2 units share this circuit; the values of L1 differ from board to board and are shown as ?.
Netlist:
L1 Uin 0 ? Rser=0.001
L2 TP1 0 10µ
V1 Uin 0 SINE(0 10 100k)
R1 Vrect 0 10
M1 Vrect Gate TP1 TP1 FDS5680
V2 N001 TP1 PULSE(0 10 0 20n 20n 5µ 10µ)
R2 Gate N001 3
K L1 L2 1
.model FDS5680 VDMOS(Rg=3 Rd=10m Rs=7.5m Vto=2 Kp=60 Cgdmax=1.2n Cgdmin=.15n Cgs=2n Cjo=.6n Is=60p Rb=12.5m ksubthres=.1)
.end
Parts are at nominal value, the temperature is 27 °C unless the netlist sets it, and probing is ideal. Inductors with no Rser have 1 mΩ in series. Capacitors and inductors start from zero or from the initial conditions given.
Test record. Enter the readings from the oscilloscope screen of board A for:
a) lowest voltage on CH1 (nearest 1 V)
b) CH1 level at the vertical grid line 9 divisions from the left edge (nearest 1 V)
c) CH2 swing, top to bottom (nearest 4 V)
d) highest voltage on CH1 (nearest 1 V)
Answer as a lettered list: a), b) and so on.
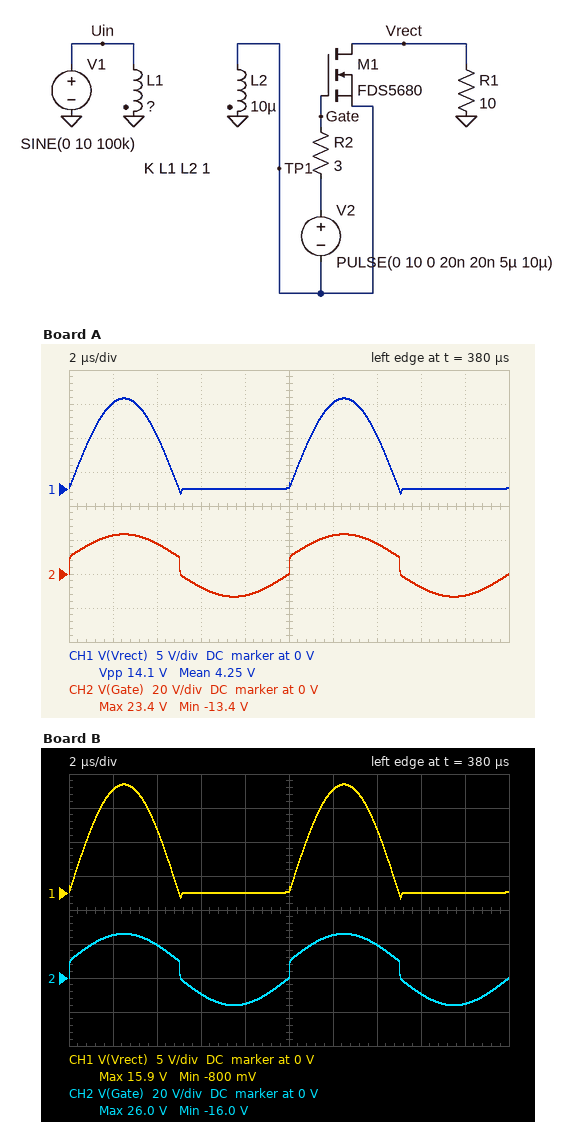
a) -1 V
b) 0 V
c) 36 V
d) 13 V
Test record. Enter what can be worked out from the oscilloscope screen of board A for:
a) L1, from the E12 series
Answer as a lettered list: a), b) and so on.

a) 5.6 µH
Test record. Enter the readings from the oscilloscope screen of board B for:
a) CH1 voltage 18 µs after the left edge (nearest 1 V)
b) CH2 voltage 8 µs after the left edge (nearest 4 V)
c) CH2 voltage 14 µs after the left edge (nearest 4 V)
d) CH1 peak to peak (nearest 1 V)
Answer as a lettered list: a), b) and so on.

a) 0 V
b) -16 V
c) 20 V
d) 17 V
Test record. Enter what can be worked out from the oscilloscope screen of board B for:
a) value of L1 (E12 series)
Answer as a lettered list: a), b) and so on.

a) 3.9 µH
